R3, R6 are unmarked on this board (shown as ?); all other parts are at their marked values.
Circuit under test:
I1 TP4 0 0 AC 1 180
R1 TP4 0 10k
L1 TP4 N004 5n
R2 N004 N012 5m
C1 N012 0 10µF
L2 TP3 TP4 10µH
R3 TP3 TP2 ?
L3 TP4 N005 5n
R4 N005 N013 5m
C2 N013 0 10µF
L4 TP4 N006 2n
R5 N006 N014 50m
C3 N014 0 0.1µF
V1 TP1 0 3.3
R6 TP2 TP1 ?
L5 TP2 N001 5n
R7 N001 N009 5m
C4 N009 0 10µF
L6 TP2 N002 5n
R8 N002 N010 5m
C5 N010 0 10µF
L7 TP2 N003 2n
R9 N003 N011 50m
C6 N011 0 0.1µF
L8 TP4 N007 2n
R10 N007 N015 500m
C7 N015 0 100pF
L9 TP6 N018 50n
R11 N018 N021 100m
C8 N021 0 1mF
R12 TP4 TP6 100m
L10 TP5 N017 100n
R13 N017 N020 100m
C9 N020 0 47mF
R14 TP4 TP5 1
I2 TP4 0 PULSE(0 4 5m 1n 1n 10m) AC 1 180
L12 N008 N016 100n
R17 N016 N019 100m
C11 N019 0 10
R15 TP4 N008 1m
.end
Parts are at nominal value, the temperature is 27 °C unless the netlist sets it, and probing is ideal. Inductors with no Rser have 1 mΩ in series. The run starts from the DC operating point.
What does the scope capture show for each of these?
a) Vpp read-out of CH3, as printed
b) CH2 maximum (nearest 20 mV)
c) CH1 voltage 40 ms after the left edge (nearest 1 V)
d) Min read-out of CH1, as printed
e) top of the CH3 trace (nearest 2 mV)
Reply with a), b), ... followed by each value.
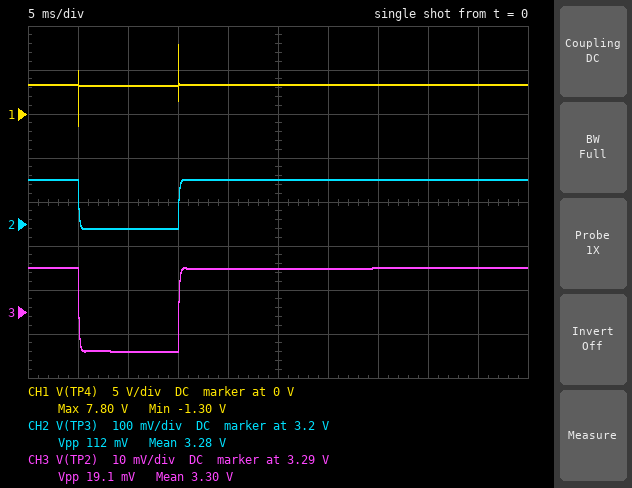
a) 19.1 mV
b) 3.30 V
c) 3 V
d) -1.30 V
e) 3.300 V
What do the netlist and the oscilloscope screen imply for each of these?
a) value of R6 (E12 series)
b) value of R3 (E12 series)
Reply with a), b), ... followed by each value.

a) 6.8 mΩ
b) 0.033 Ω
